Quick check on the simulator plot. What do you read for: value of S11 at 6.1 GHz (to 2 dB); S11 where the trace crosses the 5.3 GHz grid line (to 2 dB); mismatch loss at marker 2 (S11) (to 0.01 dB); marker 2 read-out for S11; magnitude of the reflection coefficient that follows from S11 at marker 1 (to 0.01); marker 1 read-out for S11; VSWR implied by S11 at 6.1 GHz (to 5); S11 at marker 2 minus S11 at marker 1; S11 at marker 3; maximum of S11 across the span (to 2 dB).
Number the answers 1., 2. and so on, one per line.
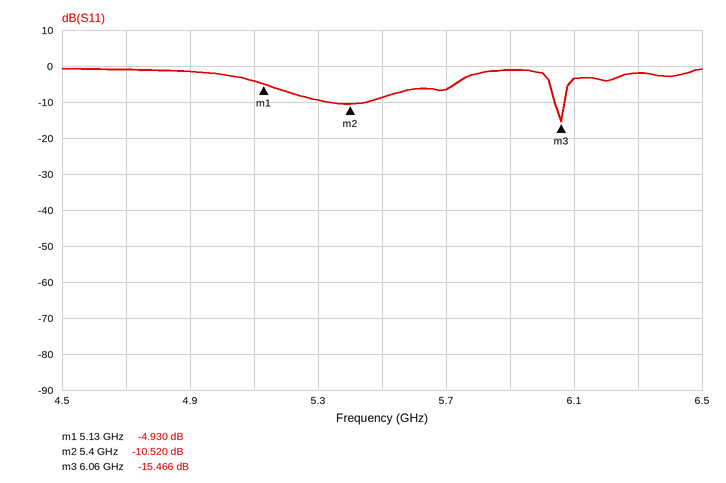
1. -4 dB
2. -10 dB
3. 0.40 dB
4. -10.520 dB
5. 0.57
6. -4.930 dB
7. 5
8. -5.590 dB
9. -15.466 dB
10. 0 dB
